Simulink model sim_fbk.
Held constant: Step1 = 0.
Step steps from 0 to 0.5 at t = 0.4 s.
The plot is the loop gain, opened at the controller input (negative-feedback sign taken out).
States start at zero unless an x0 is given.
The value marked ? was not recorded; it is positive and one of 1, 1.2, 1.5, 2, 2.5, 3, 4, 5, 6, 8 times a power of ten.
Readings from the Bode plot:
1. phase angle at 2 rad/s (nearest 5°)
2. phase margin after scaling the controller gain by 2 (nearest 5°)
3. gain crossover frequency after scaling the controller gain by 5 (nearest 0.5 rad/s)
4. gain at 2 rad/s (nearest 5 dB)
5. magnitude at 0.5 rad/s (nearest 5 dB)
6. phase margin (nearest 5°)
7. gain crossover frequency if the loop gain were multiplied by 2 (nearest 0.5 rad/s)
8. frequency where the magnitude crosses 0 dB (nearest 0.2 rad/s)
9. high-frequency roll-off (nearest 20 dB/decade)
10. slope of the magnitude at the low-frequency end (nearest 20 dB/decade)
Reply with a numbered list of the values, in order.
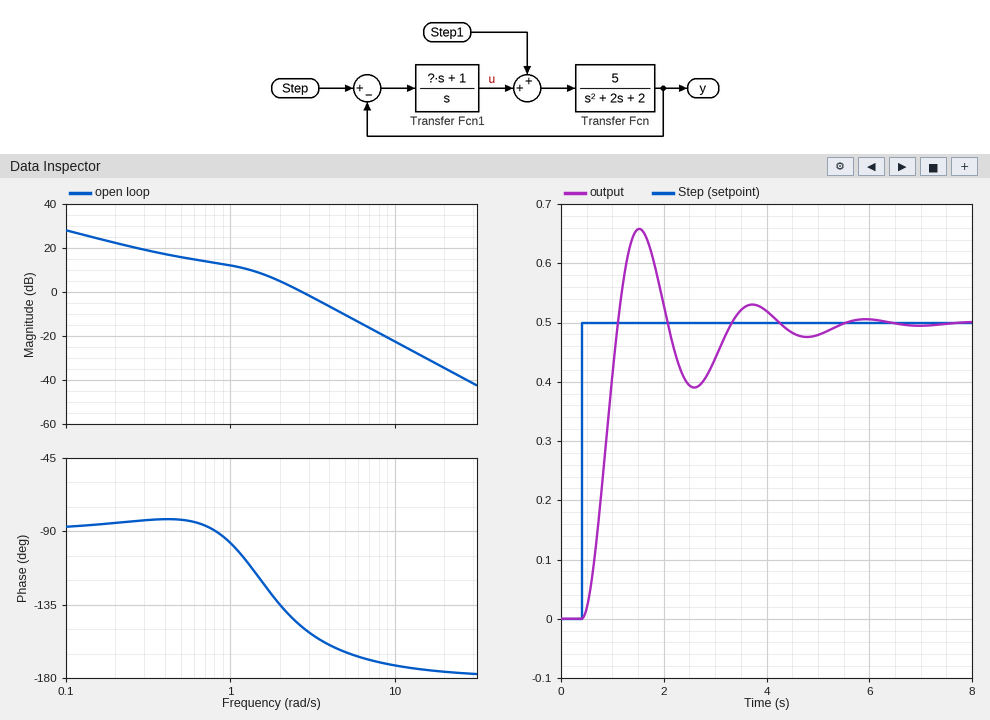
1. -135°
2. 20°
3. 6.0 rad/s
4. 5 dB
5. 15 dB
6. 30°
7. 4.0 rad/s
8. 2.8 rad/s
9. -40 dB/decade
10. -20 dB/decade
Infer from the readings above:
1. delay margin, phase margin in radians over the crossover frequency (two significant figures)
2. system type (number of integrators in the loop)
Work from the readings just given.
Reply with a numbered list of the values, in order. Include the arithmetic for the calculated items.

1. 30 × π / 180 / 2.8 = 0.19 s
2. 1
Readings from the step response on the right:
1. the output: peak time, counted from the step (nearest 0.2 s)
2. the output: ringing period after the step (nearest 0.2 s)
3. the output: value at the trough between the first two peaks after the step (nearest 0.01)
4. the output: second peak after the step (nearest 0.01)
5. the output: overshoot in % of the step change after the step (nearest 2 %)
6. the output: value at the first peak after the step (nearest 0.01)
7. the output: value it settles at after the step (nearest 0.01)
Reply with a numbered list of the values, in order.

1. 1.2 s
2. 2.2 s
3. 0.39
4. 0.53
5. 32 %
6. 0.66
7. 0.50
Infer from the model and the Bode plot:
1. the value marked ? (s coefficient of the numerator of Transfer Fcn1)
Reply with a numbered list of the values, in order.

1. 1.5
